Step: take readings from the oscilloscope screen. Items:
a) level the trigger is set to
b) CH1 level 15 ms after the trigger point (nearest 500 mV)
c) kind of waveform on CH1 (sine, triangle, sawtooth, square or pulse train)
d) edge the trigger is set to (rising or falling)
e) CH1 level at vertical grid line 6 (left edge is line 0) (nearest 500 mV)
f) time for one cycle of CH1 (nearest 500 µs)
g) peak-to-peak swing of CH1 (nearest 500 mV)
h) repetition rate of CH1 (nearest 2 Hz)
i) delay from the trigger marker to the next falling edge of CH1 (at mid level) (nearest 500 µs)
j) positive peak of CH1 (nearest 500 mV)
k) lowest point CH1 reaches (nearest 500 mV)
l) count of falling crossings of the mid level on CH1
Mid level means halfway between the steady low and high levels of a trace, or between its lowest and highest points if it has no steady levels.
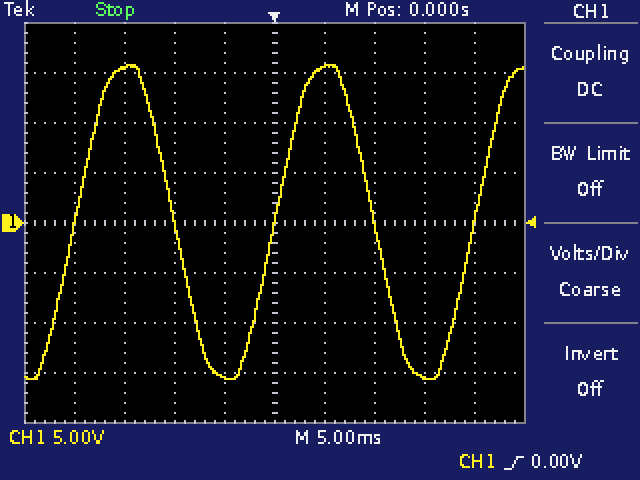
0.00 V
-15.5 V
sine
rising
15.5 V
20.0 ms
31.5 V
50 Hz
10.0 ms
16.0 V
-15.5 V
2
